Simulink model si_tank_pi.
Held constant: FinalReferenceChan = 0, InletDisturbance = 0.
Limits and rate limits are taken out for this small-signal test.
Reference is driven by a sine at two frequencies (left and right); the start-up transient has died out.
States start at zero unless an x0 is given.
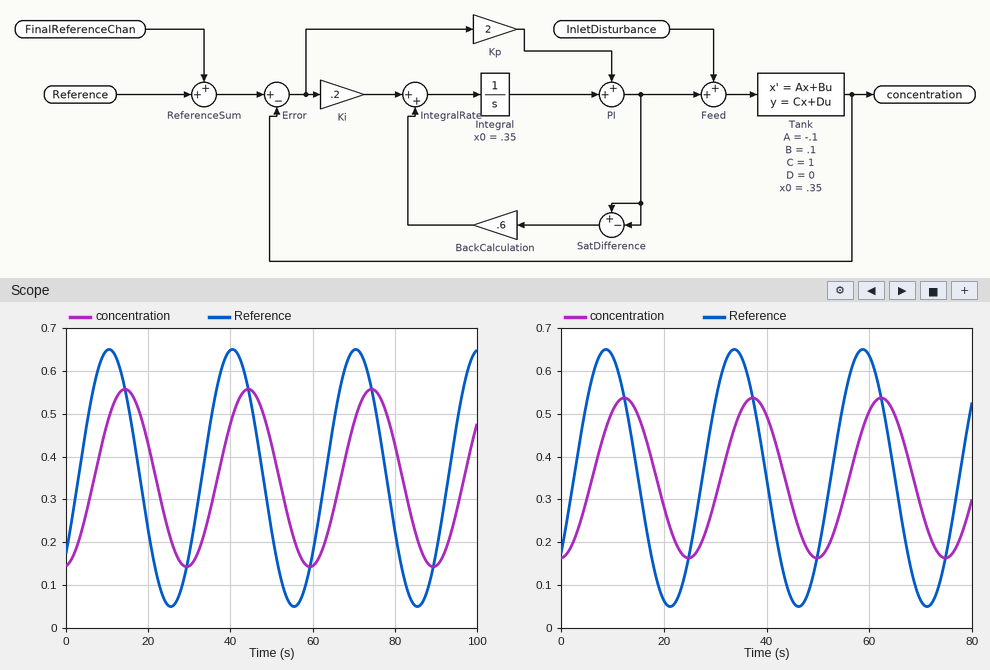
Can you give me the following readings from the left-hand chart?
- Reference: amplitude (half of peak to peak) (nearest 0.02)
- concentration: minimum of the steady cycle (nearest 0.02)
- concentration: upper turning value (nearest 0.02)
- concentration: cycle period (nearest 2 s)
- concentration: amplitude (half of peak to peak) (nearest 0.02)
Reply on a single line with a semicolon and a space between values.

0.30; 0.14; 0.56; 30 s; 0.20
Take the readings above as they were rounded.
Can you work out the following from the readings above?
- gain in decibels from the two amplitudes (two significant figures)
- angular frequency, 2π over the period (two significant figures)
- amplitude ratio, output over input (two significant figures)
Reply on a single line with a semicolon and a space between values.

-3.5 dB; 0.21 rad/s; 0.67
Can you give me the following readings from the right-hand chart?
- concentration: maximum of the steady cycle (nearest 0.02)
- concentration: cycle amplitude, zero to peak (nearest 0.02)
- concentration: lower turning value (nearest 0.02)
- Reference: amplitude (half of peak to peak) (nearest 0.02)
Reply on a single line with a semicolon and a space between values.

0.54; 0.18; 0.16; 0.30
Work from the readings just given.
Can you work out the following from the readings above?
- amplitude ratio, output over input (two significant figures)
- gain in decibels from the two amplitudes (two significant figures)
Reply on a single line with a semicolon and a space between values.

0.60; -4.4 dB
